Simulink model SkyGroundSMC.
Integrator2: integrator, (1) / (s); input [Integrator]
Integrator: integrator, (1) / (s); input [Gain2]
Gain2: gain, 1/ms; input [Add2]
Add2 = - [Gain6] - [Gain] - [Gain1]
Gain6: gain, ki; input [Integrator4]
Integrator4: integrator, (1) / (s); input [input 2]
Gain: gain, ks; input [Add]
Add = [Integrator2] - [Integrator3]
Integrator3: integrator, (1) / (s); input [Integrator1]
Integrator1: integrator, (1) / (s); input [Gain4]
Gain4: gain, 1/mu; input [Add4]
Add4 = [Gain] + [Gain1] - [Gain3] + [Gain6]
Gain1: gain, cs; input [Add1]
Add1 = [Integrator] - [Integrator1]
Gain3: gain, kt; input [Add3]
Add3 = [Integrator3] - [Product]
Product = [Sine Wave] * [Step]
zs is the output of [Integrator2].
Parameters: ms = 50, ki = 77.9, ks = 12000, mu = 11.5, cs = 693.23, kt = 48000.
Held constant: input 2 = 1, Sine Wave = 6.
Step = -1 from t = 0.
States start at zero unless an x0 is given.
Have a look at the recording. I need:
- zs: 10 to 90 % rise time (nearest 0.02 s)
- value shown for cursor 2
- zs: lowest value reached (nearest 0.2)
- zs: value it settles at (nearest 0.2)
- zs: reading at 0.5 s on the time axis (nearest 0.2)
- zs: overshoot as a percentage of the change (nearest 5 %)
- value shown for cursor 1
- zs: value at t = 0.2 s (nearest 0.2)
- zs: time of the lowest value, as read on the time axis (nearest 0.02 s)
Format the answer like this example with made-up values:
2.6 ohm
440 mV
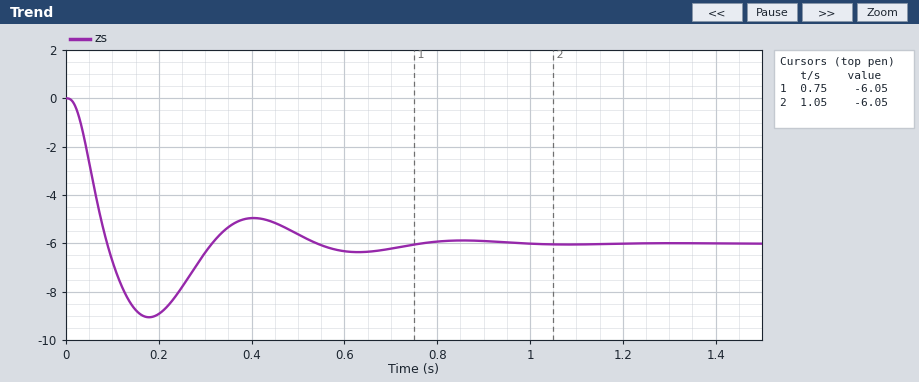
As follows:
0.06 s
-6.05
-9.0
-6.0
-5.6
50 %
-6.05
-9.0
0.18 s
